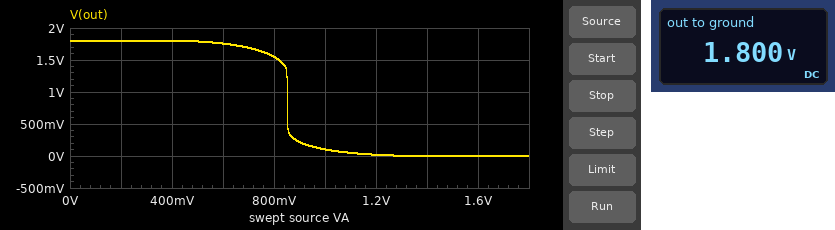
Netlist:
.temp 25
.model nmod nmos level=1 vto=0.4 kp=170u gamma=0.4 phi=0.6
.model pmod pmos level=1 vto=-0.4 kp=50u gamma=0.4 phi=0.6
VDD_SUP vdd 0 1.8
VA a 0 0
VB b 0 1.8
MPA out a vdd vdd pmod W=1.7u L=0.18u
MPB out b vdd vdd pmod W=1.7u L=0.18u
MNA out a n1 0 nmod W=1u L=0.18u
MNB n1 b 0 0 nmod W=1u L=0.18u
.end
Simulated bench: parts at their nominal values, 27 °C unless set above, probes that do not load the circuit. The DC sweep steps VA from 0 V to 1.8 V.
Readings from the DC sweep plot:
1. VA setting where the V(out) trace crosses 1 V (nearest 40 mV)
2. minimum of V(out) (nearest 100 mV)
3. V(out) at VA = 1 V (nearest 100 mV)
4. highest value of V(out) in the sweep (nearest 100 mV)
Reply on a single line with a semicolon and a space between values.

840 mV; 0 V; 100 mV; 1.8 V
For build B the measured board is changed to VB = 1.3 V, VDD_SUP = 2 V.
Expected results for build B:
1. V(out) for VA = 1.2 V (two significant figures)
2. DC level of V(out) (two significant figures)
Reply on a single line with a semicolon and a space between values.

160 mV; 2.0 V
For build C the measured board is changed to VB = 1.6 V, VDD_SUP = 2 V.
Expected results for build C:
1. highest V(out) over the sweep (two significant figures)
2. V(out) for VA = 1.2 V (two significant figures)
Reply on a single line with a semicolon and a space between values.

2.0 V; 87 mV
